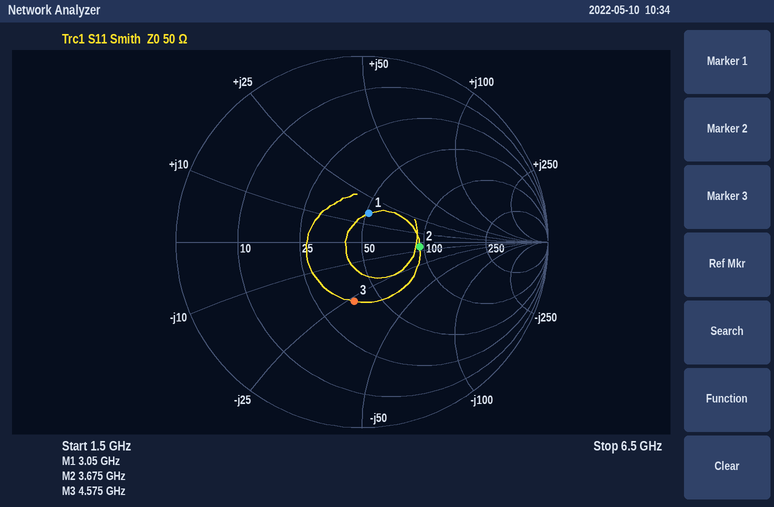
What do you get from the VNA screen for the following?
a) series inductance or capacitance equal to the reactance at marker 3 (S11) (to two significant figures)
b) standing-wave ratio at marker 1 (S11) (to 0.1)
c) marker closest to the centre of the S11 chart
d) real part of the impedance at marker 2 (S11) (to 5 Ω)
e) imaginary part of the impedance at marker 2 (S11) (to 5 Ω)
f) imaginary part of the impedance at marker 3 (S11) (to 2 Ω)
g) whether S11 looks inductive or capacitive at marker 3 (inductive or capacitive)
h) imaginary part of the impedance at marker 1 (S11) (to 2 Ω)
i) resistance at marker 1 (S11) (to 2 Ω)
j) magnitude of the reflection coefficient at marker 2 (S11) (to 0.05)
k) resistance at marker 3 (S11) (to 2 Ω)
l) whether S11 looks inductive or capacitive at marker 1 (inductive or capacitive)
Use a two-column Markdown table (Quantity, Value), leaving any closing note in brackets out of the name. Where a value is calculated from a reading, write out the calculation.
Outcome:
| Quantity | Value |
|---|---|
| series inductance or capacitance equal to the reactance at marker 3 (S11) | C = 1/(2π × 4.575 GHz × 26 Ω) ≈ 1.3 pF |
| standing-wave ratio at marker 1 (S11) | 1.4 |
| marker closest to the centre of the S11 chart | marker 1 |
| real part of the impedance at marker 2 (S11) | 95 Ω |
| imaginary part of the impedance at marker 2 (S11) | -5 Ω |
| imaginary part of the impedance at marker 3 (S11) | -26 Ω |
| whether S11 looks inductive or capacitive at marker 3 | capacitive |
| imaginary part of the impedance at marker 1 (S11) | +16 Ω |
| resistance at marker 1 (S11) | 52 Ω |
| magnitude of the reflection coefficient at marker 2 (S11) | 0.30 |
| resistance at marker 3 (S11) | 38 Ω |
| whether S11 looks inductive or capacitive at marker 1 | inductive |
